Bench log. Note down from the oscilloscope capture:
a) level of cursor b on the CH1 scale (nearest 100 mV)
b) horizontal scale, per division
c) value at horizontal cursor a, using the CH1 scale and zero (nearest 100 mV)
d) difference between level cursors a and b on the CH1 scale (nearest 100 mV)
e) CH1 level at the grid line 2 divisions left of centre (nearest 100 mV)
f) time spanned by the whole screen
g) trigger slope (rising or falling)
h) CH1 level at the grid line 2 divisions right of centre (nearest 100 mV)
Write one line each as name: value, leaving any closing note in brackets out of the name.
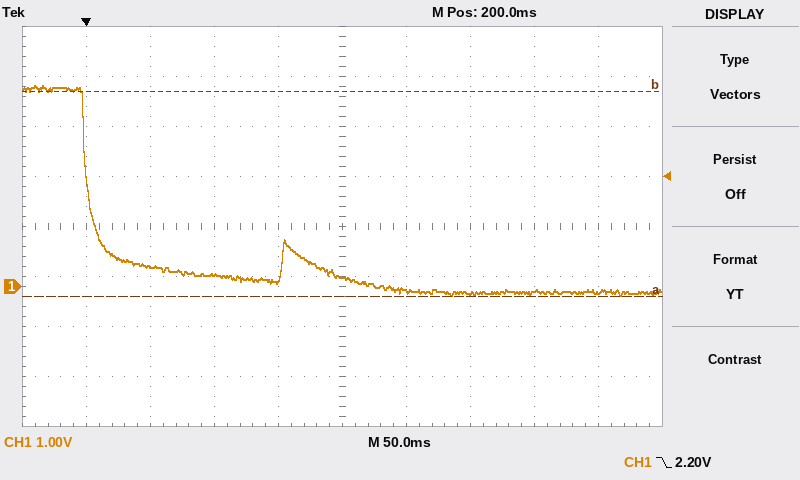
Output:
level of cursor b on the CH1 scale: 3.9 V
horizontal scale, per division: 50 ms
value at horizontal cursor a, using the CH1 scale and zero: -200 mV
difference between level cursors a and b on the CH1 scale: 4.1 V
CH1 level at the grid line 2 divisions left of centre: 200 mV
time spanned by the whole screen: 500 ms
trigger slope: falling
CH1 level at the grid line 2 divisions right of centre: -100 mV
